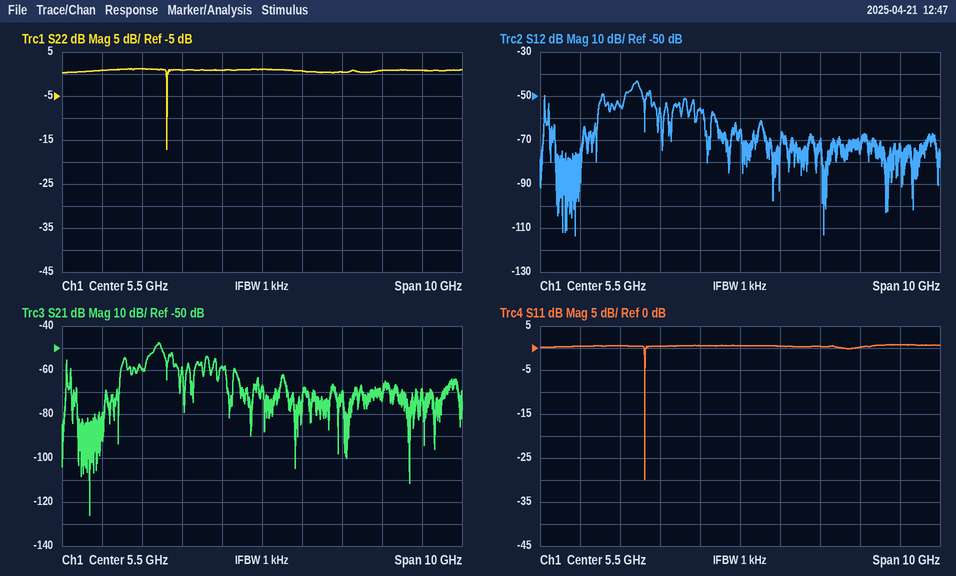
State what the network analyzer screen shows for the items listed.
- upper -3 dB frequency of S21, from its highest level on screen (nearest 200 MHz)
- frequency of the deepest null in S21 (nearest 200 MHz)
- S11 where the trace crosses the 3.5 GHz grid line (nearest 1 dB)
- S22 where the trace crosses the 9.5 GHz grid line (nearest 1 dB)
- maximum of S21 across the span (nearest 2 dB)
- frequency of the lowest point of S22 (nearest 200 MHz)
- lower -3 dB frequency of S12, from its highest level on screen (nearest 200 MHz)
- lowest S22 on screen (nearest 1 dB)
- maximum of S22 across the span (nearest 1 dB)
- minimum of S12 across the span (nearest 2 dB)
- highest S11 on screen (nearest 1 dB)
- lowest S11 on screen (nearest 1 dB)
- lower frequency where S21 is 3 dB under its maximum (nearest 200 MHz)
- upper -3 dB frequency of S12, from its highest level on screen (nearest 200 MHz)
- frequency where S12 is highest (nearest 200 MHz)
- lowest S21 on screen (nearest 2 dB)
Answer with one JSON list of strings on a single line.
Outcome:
["3.0 GHz", "1.2 GHz", "0 dB", "1 dB", "-48 dB", "3.2 GHz", "2.8 GHz", "-17 dB", "1 dB", "-114 dB", "1 dB", "-30 dB", "2.8 GHz", "3.0 GHz", "3.0 GHz", "-126 dB"]
